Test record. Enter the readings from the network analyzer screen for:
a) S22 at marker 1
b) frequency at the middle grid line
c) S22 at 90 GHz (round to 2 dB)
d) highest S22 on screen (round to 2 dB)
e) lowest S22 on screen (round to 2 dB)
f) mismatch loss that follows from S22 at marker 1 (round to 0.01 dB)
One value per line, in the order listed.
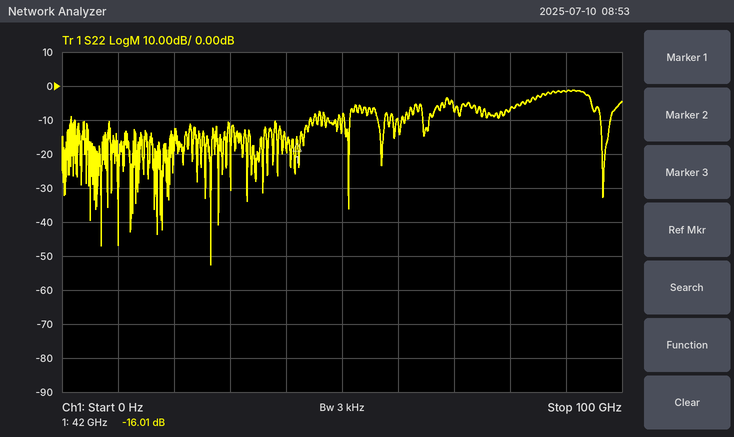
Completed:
-16.01 dB
50 GHz
-2 dB
-2 dB
-52 dB
0.11 dB
